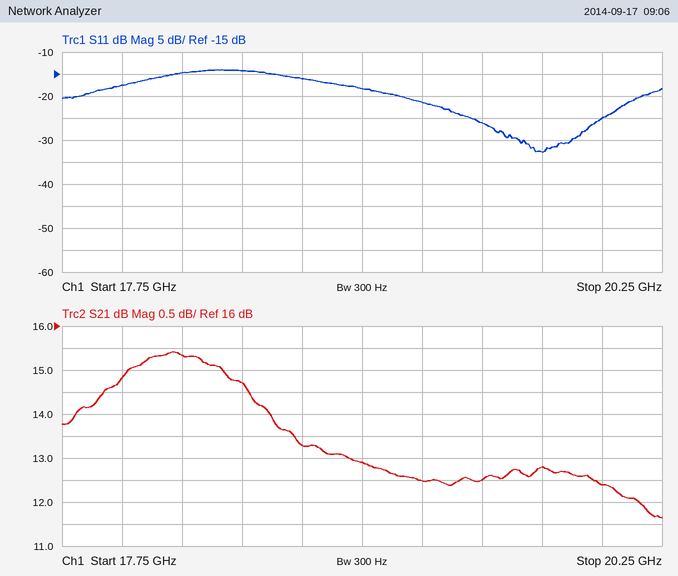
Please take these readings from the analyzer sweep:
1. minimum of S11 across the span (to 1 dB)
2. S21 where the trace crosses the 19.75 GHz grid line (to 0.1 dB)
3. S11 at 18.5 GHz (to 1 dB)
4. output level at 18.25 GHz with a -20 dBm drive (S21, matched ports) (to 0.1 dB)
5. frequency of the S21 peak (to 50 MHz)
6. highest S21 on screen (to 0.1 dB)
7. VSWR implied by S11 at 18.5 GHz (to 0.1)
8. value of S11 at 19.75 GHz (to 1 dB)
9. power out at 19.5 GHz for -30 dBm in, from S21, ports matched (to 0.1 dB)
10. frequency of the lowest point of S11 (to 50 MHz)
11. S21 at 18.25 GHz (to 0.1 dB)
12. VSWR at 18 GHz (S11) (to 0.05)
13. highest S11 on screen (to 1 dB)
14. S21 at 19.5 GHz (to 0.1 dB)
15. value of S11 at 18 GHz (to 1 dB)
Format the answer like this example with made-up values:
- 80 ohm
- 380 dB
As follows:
- -33 dB
- 12.8 dB
- -14 dB
- -4.7 dBm
- 18.20 GHz
- 15.4 dB
- 1.5
- -33 dB
- -17.5 dBm
- 19.75 GHz
- 15.3 dB
- 1.30
- -14 dB
- 12.5 dB
- -18 dB
